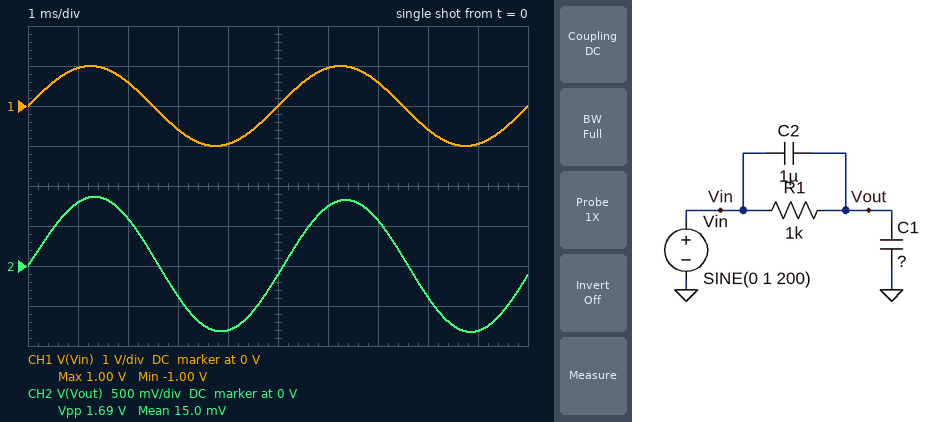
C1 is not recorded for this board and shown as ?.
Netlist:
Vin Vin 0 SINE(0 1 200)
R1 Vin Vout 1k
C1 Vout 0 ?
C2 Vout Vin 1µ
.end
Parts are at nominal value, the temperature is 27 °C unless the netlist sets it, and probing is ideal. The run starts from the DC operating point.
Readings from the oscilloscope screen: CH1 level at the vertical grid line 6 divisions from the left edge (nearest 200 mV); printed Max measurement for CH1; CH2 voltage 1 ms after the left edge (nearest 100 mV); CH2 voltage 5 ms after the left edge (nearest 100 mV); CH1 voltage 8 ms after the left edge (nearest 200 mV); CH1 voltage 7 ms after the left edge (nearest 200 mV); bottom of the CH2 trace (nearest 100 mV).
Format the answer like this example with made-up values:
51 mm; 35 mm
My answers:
1.0 V; 1.00 V; 800 mV; -100 mV; -600 mV; 600 mV; -800 mV
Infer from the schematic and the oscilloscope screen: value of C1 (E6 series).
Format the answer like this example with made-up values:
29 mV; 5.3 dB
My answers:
330 nF
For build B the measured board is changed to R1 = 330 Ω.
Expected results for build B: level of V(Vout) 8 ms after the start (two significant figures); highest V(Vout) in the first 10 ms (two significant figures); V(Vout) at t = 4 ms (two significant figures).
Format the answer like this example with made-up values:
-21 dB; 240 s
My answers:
-470 mV; 950 mV; -930 mV
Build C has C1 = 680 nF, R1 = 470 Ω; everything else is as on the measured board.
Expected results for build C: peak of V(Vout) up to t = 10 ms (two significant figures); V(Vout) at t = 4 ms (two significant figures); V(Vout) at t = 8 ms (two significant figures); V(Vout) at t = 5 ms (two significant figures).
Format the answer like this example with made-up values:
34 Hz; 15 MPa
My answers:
860 mV; -820 mV; -310 mV; -200 mV
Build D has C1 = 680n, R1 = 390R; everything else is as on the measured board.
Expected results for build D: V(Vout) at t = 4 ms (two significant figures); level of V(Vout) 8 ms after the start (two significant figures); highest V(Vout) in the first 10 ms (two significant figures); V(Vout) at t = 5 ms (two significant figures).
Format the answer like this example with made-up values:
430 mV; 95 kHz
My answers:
-860 mV; -330 mV; 880 mV; -200 mV
